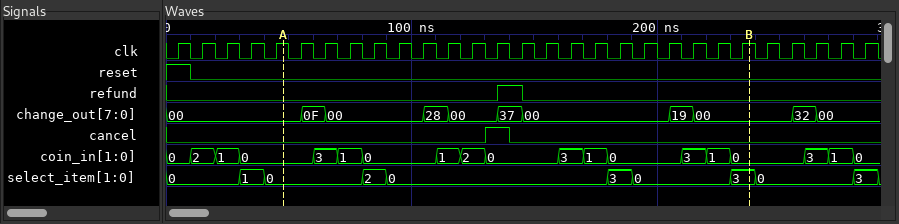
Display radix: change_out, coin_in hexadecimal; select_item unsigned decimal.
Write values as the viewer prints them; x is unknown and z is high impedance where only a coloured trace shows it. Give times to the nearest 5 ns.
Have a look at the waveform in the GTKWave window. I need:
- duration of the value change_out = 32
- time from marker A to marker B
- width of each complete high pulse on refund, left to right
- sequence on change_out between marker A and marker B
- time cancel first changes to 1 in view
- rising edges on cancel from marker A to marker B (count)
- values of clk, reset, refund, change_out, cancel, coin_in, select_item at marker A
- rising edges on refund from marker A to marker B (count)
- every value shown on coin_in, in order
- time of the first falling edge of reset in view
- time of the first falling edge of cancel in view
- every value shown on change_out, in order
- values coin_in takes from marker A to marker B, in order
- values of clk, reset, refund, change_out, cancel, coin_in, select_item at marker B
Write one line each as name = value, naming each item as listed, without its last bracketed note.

duration of the value change_out = 32 = 10 ns
time from marker A to marker B = 190 ns
width of each complete high pulse on refund, left to right = 10 ns
sequence on change_out between marker A and marker B = 00, 0F, 00, 28, 00, 37, 00, 19, 00
time cancel first changes to 1 in view = 130 ns
rising edges on cancel from marker A to marker B = 1
values of clk, reset, refund, change_out, cancel, coin_in, select_item at marker A = clk=1, reset=0, refund=0, change_out=00, cancel=0, coin_in=0, select_item=0
rising edges on refund from marker A to marker B = 1
every value shown on coin_in, in order = 0, 2, 1, 0, 3, 1, 0, 1, 2, 0, 3, 1, 0, 3, 1, 0, 3, 1, 0
time of the first falling edge of reset in view = 10 ns
time of the first falling edge of cancel in view = 140 ns
every value shown on change_out, in order = 00, 0F, 00, 28, 00, 37, 00, 19, 00, 32, 00
values coin_in takes from marker A to marker B, in order = 0, 3, 1, 0, 1, 2, 0, 3, 1, 0, 3, 1, 0
values of clk, reset, refund, change_out, cancel, coin_in, select_item at marker B = clk=1, reset=0, refund=0, change_out=00, cancel=0, coin_in=0, select_item=3
